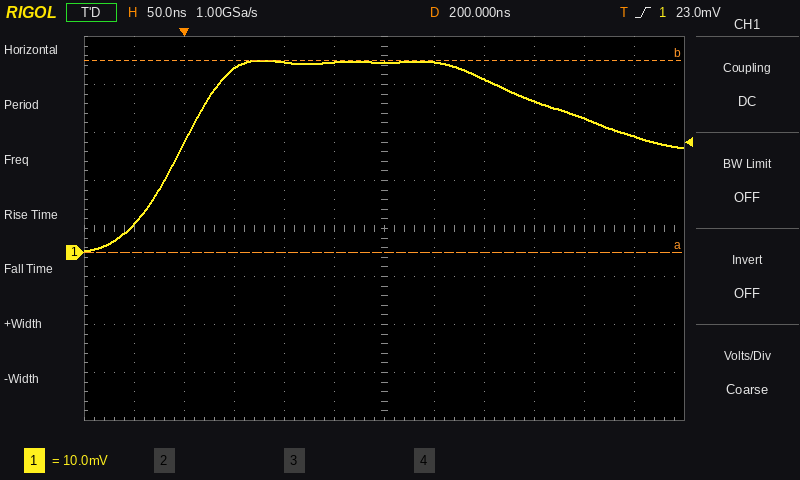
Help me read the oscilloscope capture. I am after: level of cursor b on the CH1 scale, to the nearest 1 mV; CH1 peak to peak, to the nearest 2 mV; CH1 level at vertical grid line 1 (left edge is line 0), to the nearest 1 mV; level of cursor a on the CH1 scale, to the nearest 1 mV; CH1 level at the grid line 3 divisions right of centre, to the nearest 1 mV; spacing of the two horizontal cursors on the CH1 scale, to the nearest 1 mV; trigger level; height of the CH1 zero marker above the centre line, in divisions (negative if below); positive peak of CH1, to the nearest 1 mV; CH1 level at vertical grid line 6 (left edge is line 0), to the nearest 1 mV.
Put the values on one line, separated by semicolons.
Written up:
40 mV; 40 mV; 6 mV; 0 mV; 32 mV; 40 mV; 23.0 mV; -0.5 div; 40 mV; 40 mV
